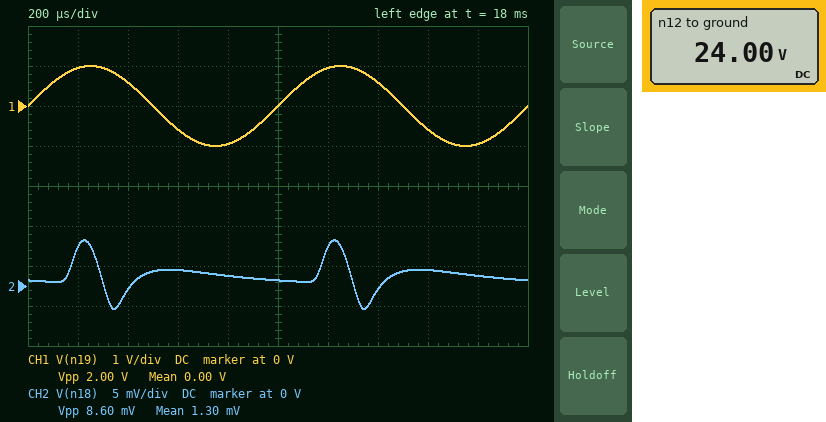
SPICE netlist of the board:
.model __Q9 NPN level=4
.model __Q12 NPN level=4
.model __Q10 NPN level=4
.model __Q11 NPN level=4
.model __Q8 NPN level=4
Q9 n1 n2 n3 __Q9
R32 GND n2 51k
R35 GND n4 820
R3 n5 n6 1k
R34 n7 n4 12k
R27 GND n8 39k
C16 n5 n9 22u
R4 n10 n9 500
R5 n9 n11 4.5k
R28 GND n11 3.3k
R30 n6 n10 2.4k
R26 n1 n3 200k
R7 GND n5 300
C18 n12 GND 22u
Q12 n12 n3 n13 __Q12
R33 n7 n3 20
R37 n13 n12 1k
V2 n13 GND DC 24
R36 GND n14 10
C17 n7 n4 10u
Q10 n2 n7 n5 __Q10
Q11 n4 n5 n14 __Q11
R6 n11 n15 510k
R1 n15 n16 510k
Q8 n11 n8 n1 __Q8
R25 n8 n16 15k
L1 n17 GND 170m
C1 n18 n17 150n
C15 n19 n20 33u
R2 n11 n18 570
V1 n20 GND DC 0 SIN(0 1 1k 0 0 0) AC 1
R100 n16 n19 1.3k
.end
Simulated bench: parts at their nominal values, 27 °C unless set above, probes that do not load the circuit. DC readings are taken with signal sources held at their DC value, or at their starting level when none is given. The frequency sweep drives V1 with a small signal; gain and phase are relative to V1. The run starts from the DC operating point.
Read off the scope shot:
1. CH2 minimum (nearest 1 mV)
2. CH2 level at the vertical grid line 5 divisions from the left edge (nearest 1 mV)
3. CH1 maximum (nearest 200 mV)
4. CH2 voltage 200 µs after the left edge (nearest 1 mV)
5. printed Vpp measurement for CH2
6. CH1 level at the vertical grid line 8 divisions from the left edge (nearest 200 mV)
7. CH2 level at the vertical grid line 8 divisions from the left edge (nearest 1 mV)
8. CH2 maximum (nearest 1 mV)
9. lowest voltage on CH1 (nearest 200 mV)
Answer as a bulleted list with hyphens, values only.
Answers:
- -3 mV
- 1 mV
- 1.0 V
- 5 mV
- 8.60 mV
- -600 mV
- 2 mV
- 6 mV
- -1.0 V
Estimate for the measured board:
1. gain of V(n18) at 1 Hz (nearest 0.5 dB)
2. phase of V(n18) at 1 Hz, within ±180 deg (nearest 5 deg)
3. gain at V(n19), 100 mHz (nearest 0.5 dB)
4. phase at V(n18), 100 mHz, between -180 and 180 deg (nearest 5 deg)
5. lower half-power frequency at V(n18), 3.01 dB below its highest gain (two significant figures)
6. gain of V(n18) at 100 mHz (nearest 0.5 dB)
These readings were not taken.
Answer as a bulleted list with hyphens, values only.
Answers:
- -53.0 dB
- 0 deg
- -2.5 dB
- 40 deg
- 88 mHz
- -55.5 dB
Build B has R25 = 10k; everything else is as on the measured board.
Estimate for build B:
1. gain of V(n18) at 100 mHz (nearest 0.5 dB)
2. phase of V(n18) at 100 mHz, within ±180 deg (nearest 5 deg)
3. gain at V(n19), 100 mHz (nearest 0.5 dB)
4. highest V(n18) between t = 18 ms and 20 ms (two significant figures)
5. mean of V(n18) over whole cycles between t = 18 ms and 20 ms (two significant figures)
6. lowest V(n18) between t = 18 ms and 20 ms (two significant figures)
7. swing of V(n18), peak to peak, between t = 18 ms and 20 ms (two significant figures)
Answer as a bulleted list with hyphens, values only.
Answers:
- -56.0 dB
- 45 deg
- -3.0 dB
- 12 mV
- 3.3 mV
- -6.0 mV
- 18 mV
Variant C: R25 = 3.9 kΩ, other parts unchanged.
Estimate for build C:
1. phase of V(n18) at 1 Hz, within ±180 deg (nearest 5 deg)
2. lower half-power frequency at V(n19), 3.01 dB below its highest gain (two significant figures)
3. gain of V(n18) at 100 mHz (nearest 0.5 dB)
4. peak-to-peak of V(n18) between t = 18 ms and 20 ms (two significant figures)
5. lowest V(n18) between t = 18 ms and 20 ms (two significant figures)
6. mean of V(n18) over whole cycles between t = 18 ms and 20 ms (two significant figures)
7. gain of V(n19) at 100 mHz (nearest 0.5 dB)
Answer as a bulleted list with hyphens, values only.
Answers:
- 5 deg
- 110 mHz
- -56.5 dB
- 49 mV
- -15 mV
- 11 mV
- -3.5 dB
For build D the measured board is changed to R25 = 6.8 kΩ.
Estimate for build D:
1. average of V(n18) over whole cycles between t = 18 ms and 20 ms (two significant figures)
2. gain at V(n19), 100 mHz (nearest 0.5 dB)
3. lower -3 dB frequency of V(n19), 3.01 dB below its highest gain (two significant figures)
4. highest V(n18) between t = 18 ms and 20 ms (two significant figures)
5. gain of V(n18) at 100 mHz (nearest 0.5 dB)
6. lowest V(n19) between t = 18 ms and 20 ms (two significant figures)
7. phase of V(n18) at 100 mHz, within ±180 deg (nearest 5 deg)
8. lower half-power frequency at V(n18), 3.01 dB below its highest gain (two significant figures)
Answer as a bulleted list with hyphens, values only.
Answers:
- 6.1 mV
- -3.5 dB
- 110 mHz
- 20 mV
- -56.0 dB
- -1.0 V
- 45 deg
- 100 mHz
